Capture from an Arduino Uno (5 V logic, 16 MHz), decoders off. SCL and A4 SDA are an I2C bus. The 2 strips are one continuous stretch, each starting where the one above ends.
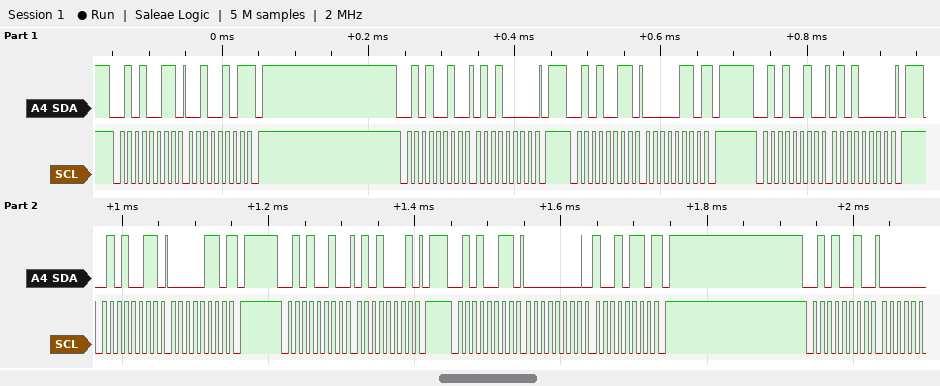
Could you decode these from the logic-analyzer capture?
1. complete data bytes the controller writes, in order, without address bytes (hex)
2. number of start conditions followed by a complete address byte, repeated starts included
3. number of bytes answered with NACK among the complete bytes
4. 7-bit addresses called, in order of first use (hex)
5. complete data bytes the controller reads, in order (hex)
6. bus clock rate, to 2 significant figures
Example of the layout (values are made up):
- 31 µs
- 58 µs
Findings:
- 50 50 51
- 8
- 4
- 0x29
- 25 06 06 00 96
- 100 kHz
